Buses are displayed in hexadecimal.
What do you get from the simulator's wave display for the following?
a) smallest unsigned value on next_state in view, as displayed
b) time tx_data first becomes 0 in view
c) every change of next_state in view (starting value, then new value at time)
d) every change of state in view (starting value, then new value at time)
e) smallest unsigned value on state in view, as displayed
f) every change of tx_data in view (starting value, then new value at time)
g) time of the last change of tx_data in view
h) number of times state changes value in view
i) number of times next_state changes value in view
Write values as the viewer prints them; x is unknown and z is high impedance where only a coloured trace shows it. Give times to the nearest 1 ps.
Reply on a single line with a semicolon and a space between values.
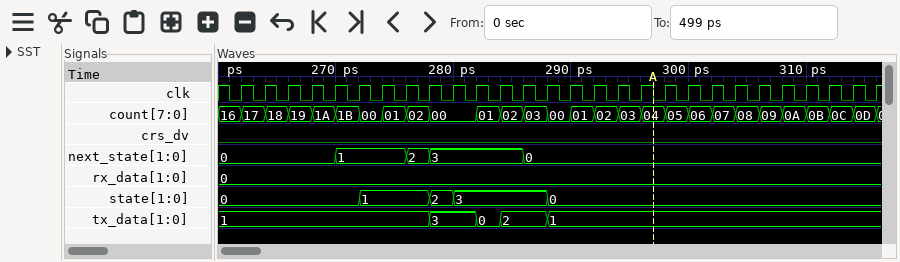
0; 282 ps; 0, 1 at 270 ps, 2 at 276 ps, 3 at 278 ps, 0 at 286 ps; 0, 1 at 272 ps, 2 at 278 ps, 3 at 280 ps, 0 at 288 ps; 0; 1, 3 at 278 ps, 0 at 282 ps, 2 at 284 ps, 1 at 288 ps; 288 ps; 4; 4
